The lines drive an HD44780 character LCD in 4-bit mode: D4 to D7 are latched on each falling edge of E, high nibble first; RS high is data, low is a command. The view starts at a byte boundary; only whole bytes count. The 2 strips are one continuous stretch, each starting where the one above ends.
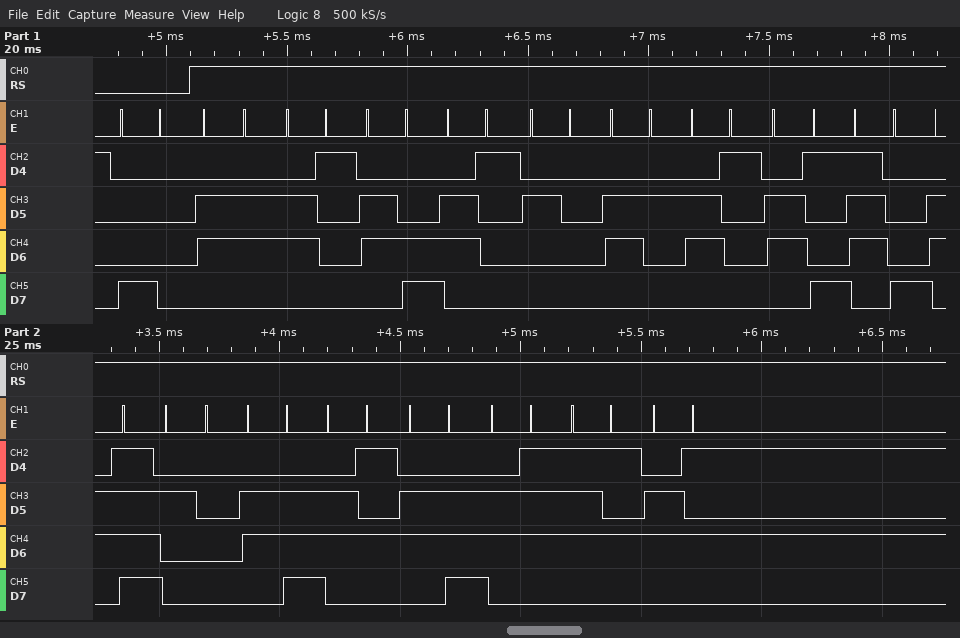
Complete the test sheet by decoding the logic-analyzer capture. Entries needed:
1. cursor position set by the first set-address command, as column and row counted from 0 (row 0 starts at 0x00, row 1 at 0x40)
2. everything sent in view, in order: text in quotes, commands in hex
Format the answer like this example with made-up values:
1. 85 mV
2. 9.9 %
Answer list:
1. column 0, row 0
2. 0x80 "fala baixo nengue"
